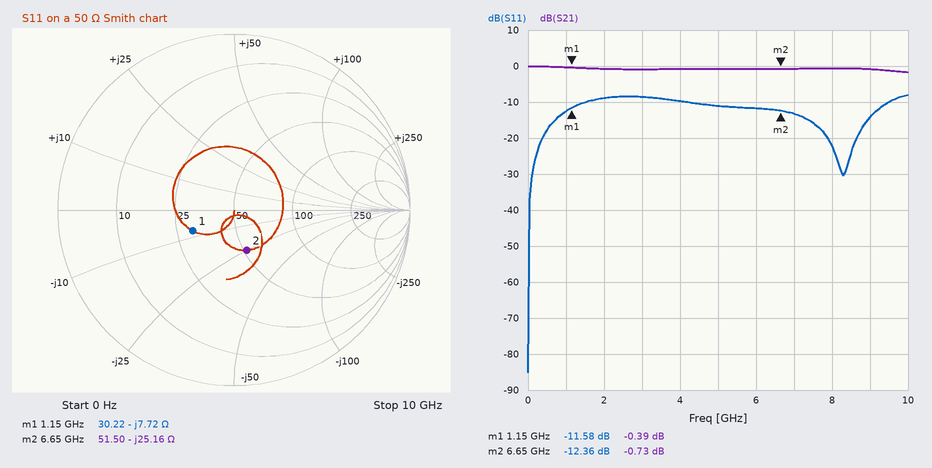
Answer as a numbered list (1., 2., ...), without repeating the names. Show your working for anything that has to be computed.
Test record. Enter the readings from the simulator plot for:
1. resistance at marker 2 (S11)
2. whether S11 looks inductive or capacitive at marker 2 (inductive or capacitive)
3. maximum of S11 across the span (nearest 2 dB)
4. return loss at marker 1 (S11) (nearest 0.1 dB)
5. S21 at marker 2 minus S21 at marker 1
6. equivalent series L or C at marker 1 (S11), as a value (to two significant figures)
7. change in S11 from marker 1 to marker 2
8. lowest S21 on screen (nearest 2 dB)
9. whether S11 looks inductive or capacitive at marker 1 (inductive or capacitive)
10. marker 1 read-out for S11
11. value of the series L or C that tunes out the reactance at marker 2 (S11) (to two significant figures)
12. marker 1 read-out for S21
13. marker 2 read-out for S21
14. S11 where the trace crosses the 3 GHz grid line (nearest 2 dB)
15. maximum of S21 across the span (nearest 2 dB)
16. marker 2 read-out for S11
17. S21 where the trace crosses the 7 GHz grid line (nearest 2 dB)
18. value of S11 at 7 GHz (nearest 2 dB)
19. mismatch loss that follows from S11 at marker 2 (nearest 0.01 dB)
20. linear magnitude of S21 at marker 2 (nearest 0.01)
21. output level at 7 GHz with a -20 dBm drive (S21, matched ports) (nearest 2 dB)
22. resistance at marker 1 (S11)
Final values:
1. 51.50 Ω
2. capacitive
3. -8 dB
4. 11.6 dB
5. -0.73 − (-0.39) = -0.34 dB
6. C = 1/(2π × 1.15 GHz × 7.72 Ω) ≈ 18 pF
7. -12.36 − (-11.58) = -0.78 dB
8. -2 dB
9. capacitive
10. -11.58 dB
11. L = 25.16 Ω/(2π × 6.65 GHz) ≈ 602 pH, so 600 pH to two significant figures
12. -0.39 dB
13. -0.73 dB
14. -8 dB
15. 0 dB
16. -12.36 dB
17. 0 dB
18. -14 dB
19. −10 log10(1 − 10^(-12.36/10)) ≈ 0.26 dB
20. 10^(-0.73/20) ≈ 0.92
21. -20 dBm + (0 dB) = -20 dBm
22. 30.22 Ω
